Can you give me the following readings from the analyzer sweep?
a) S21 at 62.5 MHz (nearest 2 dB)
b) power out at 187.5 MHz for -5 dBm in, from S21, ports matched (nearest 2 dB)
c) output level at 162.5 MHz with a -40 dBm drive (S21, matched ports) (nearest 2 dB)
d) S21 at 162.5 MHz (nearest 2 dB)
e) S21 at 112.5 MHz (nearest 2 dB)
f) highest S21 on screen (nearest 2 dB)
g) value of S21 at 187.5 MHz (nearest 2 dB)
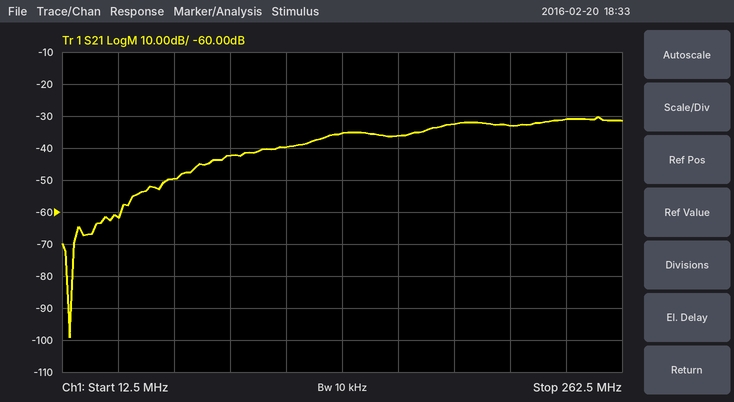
-50 dB
-38 dBm
-76 dBm
-36 dB
-40 dB
-30 dB
-32 dB
